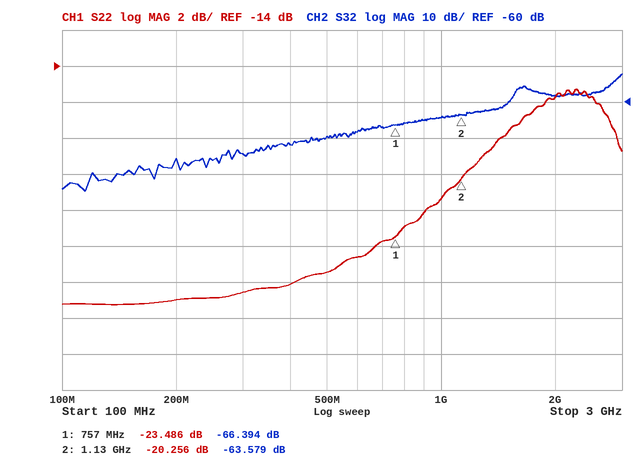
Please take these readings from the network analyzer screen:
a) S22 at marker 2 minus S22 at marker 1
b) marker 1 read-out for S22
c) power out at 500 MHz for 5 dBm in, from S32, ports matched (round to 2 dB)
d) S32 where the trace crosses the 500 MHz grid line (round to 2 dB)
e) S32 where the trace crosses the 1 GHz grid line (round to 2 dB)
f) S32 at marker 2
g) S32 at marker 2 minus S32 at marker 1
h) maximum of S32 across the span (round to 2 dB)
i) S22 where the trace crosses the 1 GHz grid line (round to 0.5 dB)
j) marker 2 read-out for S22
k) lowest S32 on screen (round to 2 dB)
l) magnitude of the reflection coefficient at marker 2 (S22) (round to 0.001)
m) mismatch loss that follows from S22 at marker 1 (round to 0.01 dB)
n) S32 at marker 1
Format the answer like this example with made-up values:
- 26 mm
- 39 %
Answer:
- 3.230 dB
- -23.486 dB
- -64 dBm
- -70 dB
- -64 dB
- -63.579 dB
- 2.815 dB
- -52 dB
- -21.5 dB
- -20.256 dB
- -84 dB
- 0.097
- 0.02 dB
- -66.394 dB
